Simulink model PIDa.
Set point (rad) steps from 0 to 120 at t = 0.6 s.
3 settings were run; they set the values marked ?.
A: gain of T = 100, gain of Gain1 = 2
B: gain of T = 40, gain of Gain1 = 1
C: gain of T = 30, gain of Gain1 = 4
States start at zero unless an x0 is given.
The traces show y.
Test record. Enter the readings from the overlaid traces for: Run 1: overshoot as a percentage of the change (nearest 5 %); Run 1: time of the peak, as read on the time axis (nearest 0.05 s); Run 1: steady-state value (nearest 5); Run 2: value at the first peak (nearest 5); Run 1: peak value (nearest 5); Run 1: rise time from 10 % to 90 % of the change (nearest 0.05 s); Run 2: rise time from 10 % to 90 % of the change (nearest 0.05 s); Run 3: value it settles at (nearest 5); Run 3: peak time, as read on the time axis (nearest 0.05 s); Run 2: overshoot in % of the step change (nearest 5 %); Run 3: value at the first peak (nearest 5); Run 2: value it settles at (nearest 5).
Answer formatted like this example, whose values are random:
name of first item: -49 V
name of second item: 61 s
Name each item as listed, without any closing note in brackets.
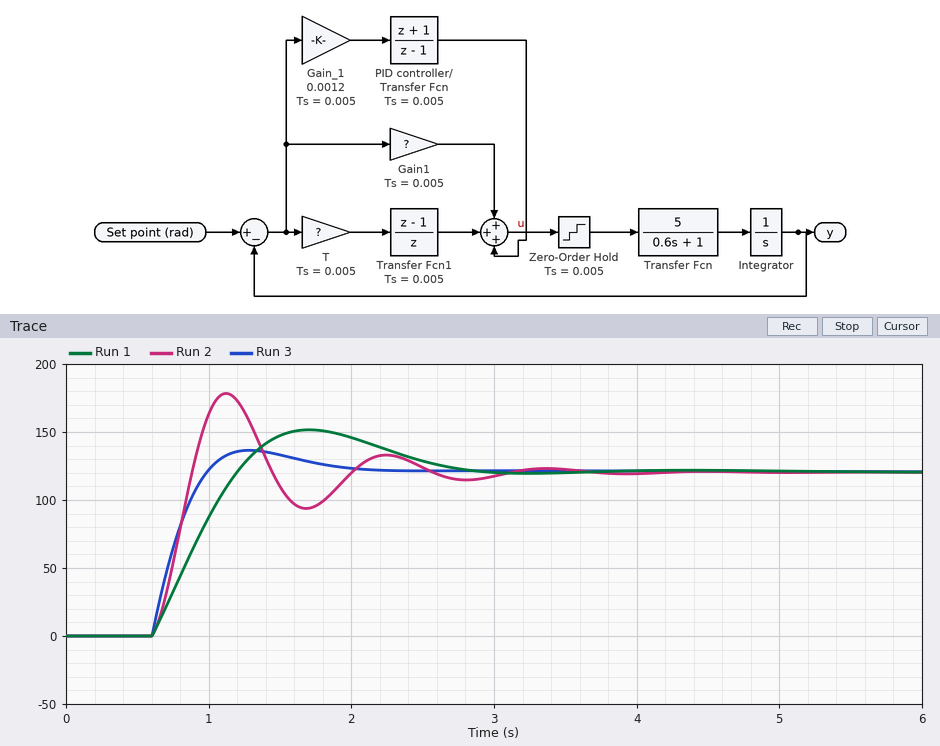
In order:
Run 1: overshoot as a percentage of the change: 25 %
Run 1: time of the peak, as read on the time axis: 1.70 s
Run 1: steady-state value: 120
Run 2: value at the first peak: 180
Run 1: peak value: 150
Run 1: rise time from 10 % to 90 % of the change: 0.45 s
Run 2: rise time from 10 % to 90 % of the change: 0.20 s
Run 3: value it settles at: 120
Run 3: peak time, as read on the time axis: 1.30 s
Run 2: overshoot in % of the step change: 50 %
Run 3: value at the first peak: 135
Run 2: value it settles at: 120
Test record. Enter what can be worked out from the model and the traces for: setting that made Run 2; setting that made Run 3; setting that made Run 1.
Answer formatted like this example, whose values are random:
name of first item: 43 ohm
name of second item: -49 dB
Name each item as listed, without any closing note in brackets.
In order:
setting that made Run 2: C
setting that made Run 3: A
setting that made Run 1: B
